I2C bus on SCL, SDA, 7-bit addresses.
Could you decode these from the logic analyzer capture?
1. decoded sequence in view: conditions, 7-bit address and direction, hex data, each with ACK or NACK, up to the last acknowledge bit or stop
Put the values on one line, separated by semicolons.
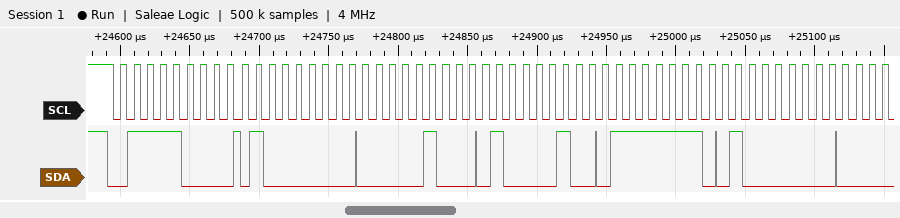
start, address 3C write ACK, 40 ACK, 04 ACK, 42 ACK, 7F ACK, 40 ACK
